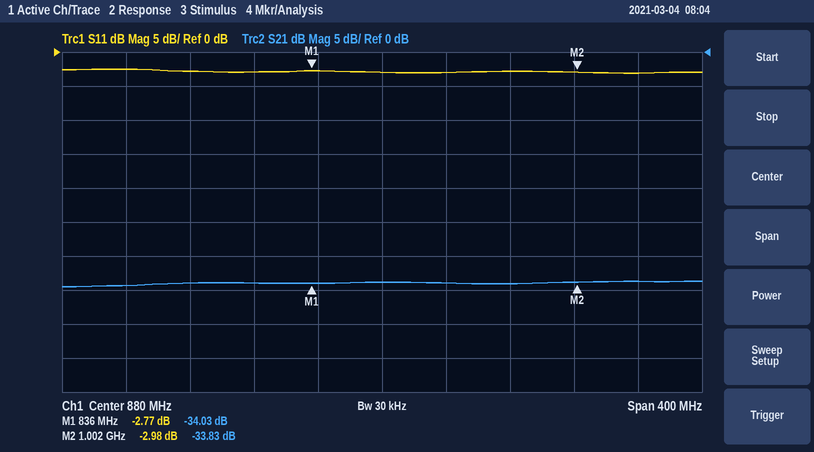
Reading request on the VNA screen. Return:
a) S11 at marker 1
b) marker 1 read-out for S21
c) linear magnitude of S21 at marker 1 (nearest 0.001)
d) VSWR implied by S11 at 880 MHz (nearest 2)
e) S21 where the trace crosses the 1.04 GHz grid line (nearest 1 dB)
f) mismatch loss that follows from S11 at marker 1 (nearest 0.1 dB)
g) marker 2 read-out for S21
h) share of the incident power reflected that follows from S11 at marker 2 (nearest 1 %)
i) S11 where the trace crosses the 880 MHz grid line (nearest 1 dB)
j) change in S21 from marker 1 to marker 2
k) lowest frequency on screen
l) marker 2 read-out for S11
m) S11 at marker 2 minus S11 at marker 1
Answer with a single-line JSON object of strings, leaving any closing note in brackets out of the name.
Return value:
{"S11 at marker 1": "-2.77 dB", "marker 1 read-out for S21": "-34.03 dB", "linear magnitude of S21 at marker 1": "0.020", "VSWR implied by S11 at 880 MHz": "6", "S21 where the trace crosses the 1.04 GHz grid line": "-34 dB", "mismatch loss that follows from S11 at marker 1": "3.3 dB", "marker 2 read-out for S21": "-33.83 dB", "share of the incident power reflected that follows from S11 at marker 2": "50 %", "S11 where the trace crosses the 880 MHz grid line": "-3 dB", "change in S21 from marker 1 to marker 2": "0.20 dB", "lowest frequency on screen": "680 MHz", "marker 2 read-out for S11": "-2.98 dB", "S11 at marker 2 minus S11 at marker 1": "-0.21 dB"}
